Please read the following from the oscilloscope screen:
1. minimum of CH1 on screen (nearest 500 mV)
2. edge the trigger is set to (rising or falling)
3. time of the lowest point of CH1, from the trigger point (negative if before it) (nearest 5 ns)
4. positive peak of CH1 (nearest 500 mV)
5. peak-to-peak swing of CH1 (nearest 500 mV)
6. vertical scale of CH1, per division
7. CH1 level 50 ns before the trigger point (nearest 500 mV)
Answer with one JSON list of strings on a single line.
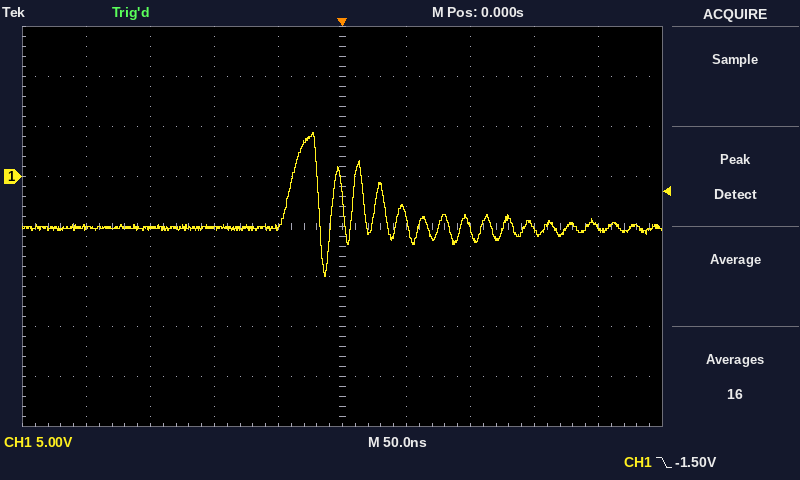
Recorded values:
["-10.0 V", "falling", "-15 ns", "4.5 V", "14.5 V", "5 V", "-5.0 V"]
